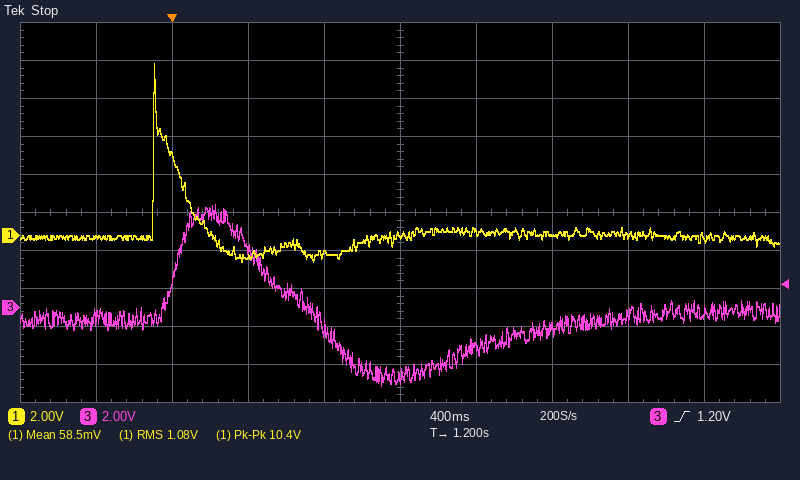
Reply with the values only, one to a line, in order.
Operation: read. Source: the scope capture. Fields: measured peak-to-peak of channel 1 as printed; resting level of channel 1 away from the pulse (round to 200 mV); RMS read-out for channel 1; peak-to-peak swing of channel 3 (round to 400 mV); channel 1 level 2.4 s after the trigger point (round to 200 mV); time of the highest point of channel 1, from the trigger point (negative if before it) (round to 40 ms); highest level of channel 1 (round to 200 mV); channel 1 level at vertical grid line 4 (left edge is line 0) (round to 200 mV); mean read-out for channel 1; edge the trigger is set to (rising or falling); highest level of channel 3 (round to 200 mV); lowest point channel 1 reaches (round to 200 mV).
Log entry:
10.4 V
0.0 V
1.08 V
9.6 V
0.0 V
-80 ms
9.0 V
-1.0 V
58.5 mV
rising
5.4 V
-1.4 V
